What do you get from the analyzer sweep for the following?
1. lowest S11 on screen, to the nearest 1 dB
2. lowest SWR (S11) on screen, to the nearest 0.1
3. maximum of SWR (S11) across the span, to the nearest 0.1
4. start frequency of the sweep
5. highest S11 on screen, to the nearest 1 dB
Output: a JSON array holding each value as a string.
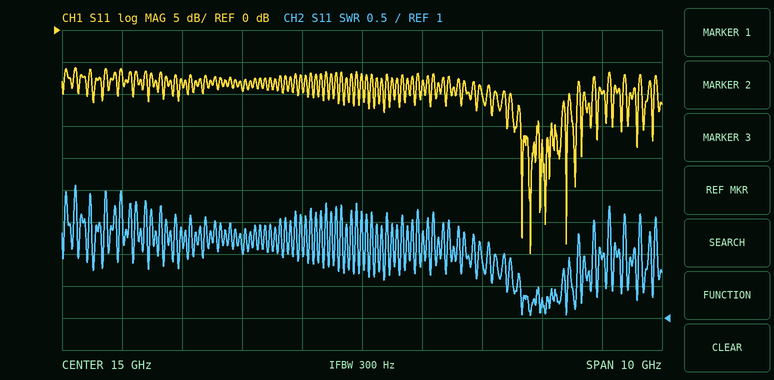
["-35 dB", "1.0", "3.1", "10 GHz", "-6 dB"]
